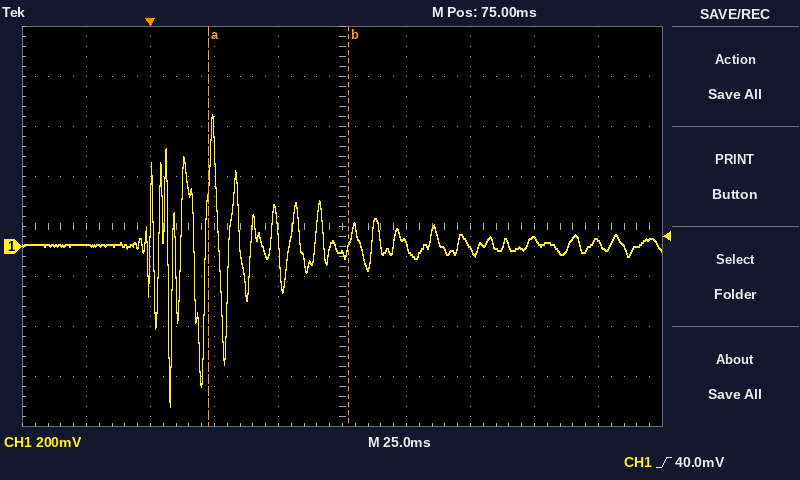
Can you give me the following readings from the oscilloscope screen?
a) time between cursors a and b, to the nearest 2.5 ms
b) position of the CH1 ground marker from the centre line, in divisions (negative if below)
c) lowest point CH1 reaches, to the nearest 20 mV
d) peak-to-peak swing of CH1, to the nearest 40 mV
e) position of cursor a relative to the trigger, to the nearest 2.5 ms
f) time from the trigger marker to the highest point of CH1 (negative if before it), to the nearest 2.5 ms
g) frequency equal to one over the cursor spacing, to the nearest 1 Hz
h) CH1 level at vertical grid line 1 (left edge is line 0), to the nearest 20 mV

55.0 ms
-0.4 div
-640 mV
1.16 V
+22.5 ms
+25.0 ms
18 Hz
0 mV
